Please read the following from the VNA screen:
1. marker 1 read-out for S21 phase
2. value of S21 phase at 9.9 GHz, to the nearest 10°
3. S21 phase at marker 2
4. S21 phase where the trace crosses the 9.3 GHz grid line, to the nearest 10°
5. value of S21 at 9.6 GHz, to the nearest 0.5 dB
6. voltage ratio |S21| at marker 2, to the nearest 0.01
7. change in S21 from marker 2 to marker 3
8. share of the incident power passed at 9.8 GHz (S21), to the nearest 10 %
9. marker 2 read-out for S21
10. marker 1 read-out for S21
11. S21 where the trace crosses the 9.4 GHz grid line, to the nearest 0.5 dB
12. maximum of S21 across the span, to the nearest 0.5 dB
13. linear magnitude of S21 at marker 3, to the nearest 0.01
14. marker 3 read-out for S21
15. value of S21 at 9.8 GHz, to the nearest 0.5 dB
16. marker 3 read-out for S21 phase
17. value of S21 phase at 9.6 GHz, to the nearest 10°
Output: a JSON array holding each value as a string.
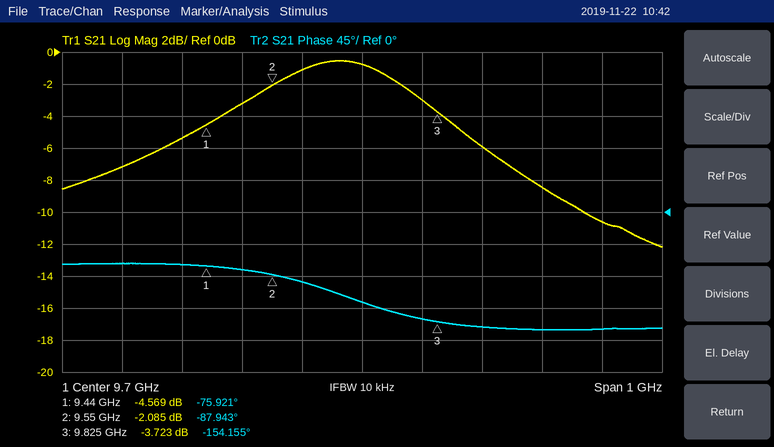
["-75.921°", "-160°", "-87.943°", "-70°", "-1.0 dB", "0.79", "-1.638 dB", "50 %", "-2.085 dB", "-4.569 dB", "-5.5 dB", "-0.5 dB", "0.65", "-3.723 dB", "-3.0 dB", "-154.155°", "-100°"]
